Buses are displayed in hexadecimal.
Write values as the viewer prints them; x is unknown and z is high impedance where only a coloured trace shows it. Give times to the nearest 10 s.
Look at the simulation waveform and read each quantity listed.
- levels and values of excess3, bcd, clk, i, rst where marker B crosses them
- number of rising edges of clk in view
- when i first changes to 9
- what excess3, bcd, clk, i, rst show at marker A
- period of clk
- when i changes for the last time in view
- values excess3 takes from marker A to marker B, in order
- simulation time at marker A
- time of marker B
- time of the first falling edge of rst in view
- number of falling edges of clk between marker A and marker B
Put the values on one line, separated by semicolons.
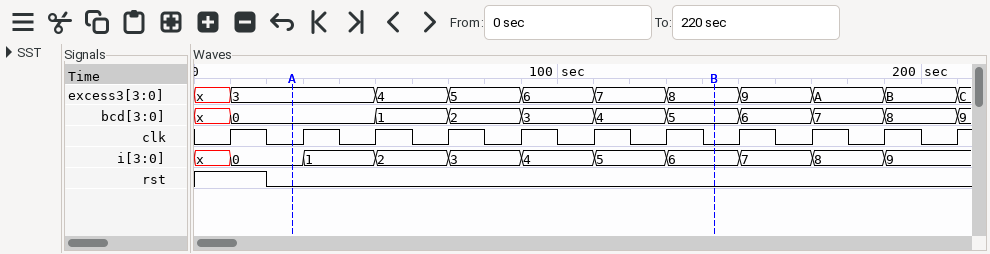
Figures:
excess3=8, bcd=5, clk=0, i=6, rst=0; 11; 190 s; excess3=3, bcd=0, clk=0, i=0, rst=0; 20 s; 190 s; 3, 4, 5, 6, 7, 8; 30 s; 140 s; 20 s; 6
